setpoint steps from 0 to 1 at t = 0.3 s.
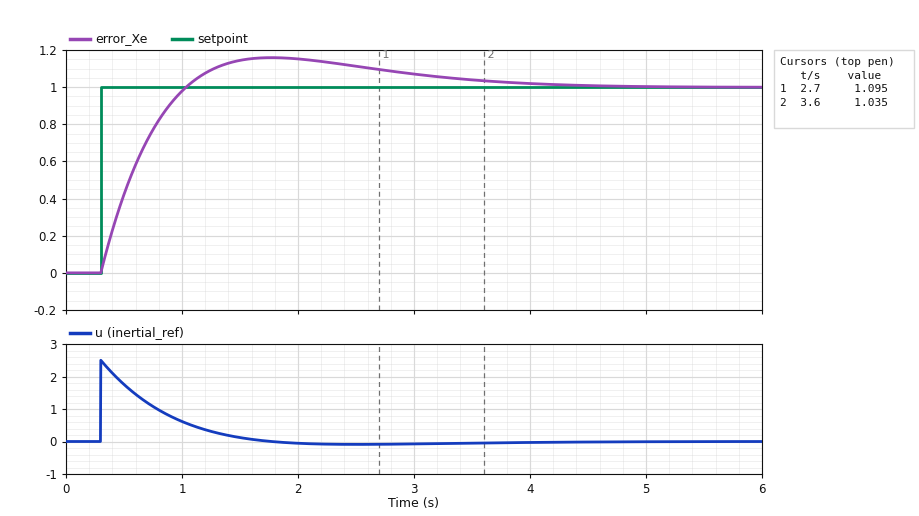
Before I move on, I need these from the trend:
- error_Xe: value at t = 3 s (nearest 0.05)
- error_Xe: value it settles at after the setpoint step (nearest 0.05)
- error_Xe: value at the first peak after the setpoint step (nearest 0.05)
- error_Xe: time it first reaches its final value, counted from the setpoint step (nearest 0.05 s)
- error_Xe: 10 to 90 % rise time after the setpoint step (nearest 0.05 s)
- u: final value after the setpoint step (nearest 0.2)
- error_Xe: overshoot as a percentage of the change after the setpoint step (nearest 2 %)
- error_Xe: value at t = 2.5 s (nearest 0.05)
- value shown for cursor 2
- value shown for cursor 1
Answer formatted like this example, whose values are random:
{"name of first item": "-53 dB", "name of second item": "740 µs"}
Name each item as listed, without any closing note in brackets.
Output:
{"error_Xe: value at t = 3 s": "1.05", "error_Xe: value it settles at after the setpoint step": "1.00", "error_Xe: value at the first peak after the setpoint step": "1.15", "error_Xe: time it first reaches its final value, counted from the setpoint step": "0.75 s", "error_Xe: 10 to 90 % rise time after the setpoint step": "0.55 s", "u: final value after the setpoint step": "0.0", "error_Xe: overshoot as a percentage of the change after the setpoint step": "16 %", "error_Xe: value at t = 2.5 s": "1.10", "value shown for cursor 2": "1.035", "value shown for cursor 1": "1.095"}
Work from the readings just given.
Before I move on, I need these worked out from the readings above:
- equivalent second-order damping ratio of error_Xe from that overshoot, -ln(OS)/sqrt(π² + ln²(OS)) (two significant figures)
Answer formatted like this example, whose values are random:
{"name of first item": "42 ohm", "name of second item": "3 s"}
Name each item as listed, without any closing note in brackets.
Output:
{"equivalent second-order damping ratio of error_Xe from that overshoot, -ln(OS)/sqrt(π² + ln²(OS))": "0.50"}
